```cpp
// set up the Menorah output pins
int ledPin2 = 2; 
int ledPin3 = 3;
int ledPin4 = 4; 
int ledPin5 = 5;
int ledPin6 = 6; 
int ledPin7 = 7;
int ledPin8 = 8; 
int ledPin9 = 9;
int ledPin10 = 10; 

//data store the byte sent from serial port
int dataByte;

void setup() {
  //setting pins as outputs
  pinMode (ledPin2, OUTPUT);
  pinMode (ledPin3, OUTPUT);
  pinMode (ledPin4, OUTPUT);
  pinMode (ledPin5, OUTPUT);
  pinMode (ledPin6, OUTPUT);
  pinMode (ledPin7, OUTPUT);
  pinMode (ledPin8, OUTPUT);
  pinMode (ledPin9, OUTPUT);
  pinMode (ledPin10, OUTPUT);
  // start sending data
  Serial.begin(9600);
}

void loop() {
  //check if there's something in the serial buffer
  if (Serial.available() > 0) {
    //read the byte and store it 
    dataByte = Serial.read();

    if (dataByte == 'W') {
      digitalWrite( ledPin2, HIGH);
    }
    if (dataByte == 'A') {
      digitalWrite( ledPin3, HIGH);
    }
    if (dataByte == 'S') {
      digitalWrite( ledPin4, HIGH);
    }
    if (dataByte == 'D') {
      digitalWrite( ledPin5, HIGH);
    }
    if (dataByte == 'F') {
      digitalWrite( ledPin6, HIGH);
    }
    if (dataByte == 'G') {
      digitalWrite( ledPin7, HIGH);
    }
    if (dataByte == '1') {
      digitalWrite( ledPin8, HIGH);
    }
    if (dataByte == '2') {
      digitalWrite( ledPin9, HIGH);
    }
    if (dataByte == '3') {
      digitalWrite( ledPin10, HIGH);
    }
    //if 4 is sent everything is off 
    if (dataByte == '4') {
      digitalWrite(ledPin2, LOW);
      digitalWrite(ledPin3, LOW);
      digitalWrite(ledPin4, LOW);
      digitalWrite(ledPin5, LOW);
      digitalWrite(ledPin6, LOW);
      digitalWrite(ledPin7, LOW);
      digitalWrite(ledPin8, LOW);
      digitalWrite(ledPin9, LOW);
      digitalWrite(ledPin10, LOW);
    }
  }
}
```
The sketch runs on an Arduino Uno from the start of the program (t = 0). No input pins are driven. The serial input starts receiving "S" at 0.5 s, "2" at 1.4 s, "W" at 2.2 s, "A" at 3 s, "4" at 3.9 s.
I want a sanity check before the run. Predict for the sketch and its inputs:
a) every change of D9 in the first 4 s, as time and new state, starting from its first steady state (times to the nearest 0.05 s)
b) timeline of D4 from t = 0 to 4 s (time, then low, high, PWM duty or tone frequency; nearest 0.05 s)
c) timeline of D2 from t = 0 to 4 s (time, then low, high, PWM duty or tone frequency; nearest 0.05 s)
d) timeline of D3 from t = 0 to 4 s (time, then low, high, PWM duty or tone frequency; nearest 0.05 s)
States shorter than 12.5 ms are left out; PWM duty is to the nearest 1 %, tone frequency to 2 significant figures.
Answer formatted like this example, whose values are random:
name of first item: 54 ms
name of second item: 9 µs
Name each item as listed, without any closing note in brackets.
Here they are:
every change of D9 in the first 4 s, as time and new state, starting from its first steady state: 0 s low; 1.4 s high; 3.9 s low
timeline of D4 from t = 0 to 4 s: 0 s low; 0.5 s high; 3.9 s low
timeline of D2 from t = 0 to 4 s: 0 s low; 2.2 s high; 3.9 s low
timeline of D3 from t = 0 to 4 s: 0 s low; 3 s high; 3.9 s low
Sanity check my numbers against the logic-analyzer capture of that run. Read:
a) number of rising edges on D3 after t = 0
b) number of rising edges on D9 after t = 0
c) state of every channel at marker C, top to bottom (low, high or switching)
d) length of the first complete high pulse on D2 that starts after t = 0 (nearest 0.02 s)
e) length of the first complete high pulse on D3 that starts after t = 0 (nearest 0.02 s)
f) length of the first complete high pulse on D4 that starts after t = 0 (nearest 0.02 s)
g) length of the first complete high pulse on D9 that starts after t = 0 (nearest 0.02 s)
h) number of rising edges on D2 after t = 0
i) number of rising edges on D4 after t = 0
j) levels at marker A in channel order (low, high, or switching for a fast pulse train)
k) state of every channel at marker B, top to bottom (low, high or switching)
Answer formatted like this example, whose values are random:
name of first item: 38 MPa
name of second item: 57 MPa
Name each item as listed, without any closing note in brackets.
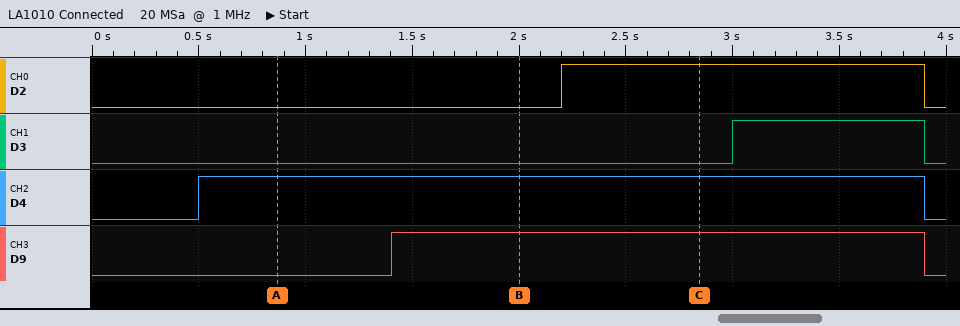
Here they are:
number of rising edges on D3 after t = 0: 1
number of rising edges on D9 after t = 0: 1
state of every channel at marker C, top to bottom: D2 high, D3 low, D4 high, D9 high
length of the first complete high pulse on D2 that starts after t = 0: 1.70 s
length of the first complete high pulse on D3 that starts after t = 0: 0.90 s
length of the first complete high pulse on D4 that starts after t = 0: 3.40 s
length of the first complete high pulse on D9 that starts after t = 0: 2.50 s
number of rising edges on D2 after t = 0: 1
number of rising edges on D4 after t = 0: 1
levels at marker A in channel order: D2 low, D3 low, D4 high, D9 low
state of every channel at marker B, top to bottom: D2 low, D3 low, D4 high, D9 high
